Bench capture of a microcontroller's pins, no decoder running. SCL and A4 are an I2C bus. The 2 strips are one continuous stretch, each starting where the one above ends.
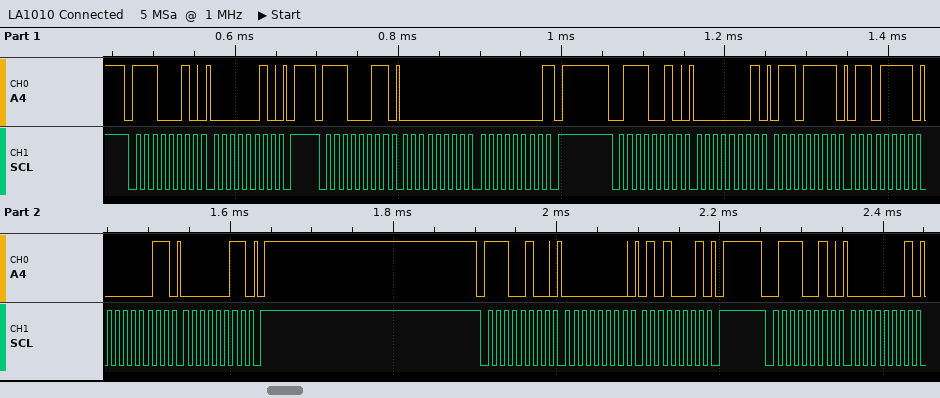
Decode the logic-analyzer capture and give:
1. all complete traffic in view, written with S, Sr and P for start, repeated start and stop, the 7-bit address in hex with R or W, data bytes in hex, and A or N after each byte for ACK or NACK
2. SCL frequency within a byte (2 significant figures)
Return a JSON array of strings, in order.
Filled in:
["S 71W A 02 A P S 71R A 00 A 00 N P S 39W A 01 A 6F A 6F A 03 A 03 A P S 72W A 00 A 51 A P S 39W A 01 A", "100 kHz"]
